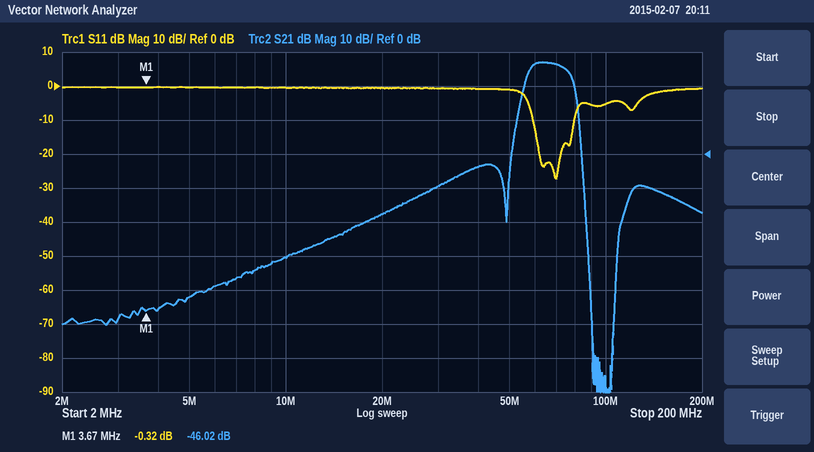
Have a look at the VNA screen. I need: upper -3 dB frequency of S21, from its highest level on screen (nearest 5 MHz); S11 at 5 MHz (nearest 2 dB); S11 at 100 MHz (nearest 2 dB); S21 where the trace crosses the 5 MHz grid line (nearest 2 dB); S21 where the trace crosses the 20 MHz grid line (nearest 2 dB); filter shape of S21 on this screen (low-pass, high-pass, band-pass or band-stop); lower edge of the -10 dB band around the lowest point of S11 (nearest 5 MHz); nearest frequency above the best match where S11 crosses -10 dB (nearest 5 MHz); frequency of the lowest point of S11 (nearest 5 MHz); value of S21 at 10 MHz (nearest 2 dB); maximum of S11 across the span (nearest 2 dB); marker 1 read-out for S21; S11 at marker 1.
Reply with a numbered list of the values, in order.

1. 75 MHz
2. 0 dB
3. -6 dB
4. -42 dB
5. -18 dB
6. band-pass
7. 60 MHz
8. 80 MHz
9. 70 MHz
10. -30 dB
11. 0 dB
12. -46.02 dB
13. -0.32 dB
